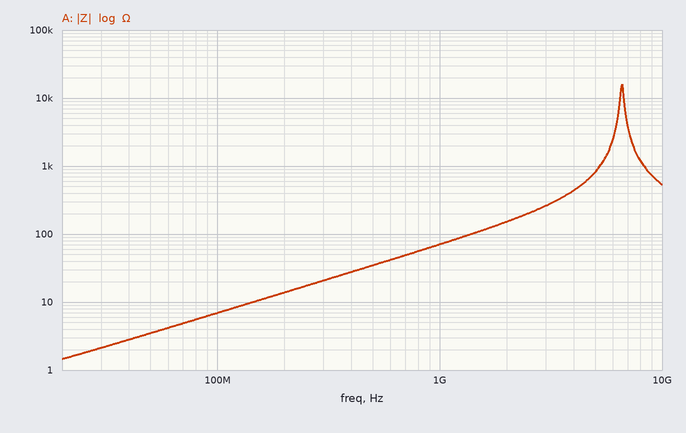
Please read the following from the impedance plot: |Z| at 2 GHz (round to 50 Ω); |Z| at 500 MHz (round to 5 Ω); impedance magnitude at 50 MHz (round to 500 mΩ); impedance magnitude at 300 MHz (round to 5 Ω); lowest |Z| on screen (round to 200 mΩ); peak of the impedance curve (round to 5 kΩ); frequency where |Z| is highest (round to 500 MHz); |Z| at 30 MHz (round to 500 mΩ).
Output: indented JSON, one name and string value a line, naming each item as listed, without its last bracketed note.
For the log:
{
  "|Z| at 2 GHz": "150 Ω",
  "|Z| at 500 MHz": "35 Ω",
  "impedance magnitude at 50 MHz": "3.5 Ω",
  "impedance magnitude at 300 MHz": "20 Ω",
  "lowest |Z| on screen": "1.4 Ω",
  "peak of the impedance curve": "15 kΩ",
  "frequency where |Z| is highest": "6.5 GHz",
  "|Z| at 30 MHz": "2.0 Ω"
}
